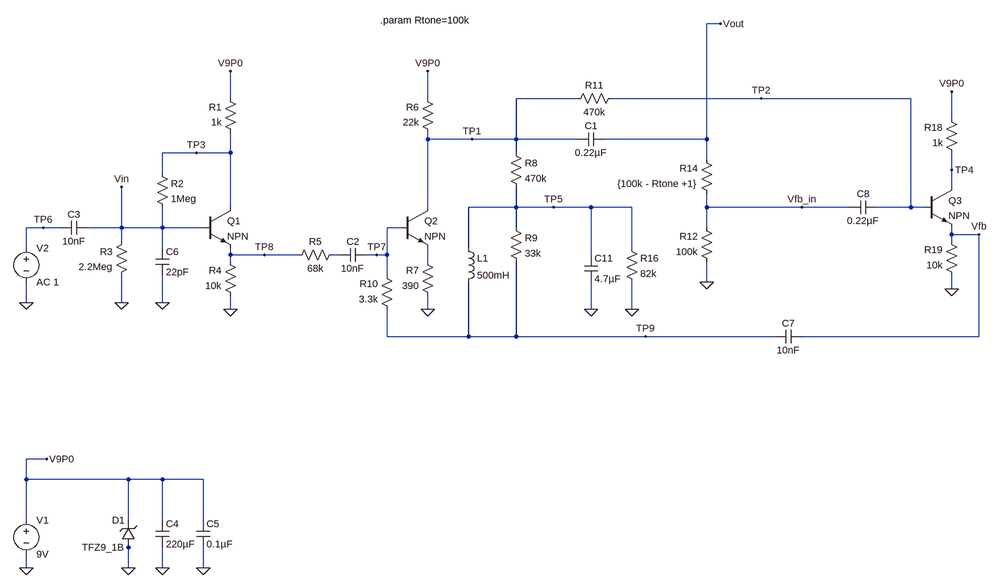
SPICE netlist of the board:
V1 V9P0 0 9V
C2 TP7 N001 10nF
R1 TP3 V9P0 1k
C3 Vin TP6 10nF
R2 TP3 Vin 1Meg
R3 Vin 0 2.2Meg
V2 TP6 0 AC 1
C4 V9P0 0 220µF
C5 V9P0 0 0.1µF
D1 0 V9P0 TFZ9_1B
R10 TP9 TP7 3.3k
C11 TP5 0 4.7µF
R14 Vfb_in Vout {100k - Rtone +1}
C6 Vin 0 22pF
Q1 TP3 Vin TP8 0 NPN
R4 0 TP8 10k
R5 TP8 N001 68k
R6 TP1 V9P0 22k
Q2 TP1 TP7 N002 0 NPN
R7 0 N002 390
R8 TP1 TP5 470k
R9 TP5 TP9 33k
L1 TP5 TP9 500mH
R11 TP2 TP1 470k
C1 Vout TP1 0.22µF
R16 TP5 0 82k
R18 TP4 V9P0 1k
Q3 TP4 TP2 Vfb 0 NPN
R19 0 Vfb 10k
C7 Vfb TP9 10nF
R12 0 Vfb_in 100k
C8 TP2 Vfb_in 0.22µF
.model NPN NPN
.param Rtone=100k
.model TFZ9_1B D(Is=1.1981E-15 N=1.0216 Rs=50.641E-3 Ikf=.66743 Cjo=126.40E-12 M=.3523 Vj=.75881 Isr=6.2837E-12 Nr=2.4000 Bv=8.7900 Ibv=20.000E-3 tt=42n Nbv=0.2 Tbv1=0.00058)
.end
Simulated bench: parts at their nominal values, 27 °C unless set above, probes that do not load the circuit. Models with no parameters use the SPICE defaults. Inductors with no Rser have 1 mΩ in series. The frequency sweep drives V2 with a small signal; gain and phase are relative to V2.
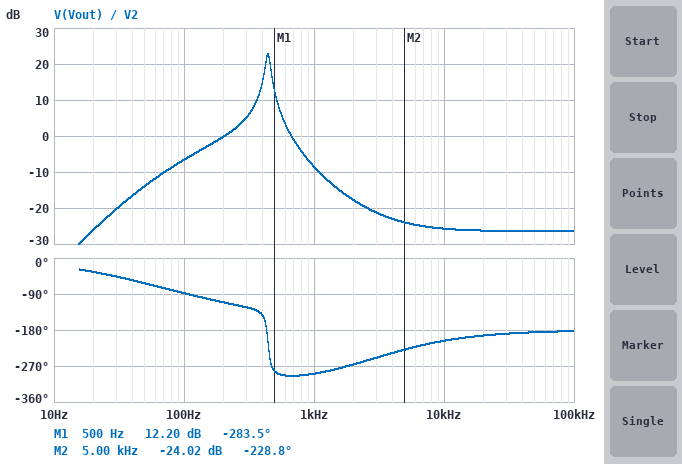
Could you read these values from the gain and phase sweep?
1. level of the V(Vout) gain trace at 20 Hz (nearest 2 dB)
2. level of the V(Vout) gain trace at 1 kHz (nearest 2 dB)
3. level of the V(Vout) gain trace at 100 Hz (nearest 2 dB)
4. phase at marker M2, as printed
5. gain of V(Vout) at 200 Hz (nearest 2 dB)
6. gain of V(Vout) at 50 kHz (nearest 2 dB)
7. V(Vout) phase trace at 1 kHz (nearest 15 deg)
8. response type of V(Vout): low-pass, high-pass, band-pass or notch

-26 dB
-8 dB
-6 dB
-228.8 deg
0 dB
-26 dB
-285 deg
band-pass
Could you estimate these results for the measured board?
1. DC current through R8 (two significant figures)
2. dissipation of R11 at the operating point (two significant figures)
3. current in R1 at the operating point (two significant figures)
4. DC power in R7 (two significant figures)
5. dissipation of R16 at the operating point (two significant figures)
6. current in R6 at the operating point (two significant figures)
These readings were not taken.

11 µA
5.6 µW
310 µA
6.7 µW
7.4 µW
140 µA
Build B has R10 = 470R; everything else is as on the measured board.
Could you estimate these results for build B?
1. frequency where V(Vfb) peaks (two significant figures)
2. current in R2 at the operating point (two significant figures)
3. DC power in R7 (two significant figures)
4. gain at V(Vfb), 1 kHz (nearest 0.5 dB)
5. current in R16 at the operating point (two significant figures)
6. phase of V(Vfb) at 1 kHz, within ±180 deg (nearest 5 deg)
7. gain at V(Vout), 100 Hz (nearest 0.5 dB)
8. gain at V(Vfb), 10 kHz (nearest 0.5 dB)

430 Hz
4.8 µA
6.8 µW
-11.5 dB
9.4 µA
100 deg
-23.0 dB
-32.5 dB
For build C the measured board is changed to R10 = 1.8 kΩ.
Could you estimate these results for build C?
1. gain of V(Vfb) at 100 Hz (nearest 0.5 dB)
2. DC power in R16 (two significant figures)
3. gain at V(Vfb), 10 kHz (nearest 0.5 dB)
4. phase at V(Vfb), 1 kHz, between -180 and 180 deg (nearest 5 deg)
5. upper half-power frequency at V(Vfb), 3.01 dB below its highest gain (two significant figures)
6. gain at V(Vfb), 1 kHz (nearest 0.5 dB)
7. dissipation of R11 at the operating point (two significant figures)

-11.5 dB
7.3 µW
-29.5 dB
85 deg
450 Hz
-10.5 dB
5.5 µW
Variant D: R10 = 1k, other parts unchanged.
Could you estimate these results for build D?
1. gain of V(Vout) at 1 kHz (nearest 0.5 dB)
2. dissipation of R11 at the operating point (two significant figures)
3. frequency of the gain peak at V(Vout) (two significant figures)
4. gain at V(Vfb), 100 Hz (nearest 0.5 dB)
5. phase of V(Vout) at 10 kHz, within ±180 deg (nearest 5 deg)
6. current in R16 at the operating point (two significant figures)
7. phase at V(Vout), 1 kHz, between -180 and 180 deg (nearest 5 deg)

-11.0 dB
5.5 µW
430 Hz
-16.5 dB
125 deg
9.4 µA
95 deg
